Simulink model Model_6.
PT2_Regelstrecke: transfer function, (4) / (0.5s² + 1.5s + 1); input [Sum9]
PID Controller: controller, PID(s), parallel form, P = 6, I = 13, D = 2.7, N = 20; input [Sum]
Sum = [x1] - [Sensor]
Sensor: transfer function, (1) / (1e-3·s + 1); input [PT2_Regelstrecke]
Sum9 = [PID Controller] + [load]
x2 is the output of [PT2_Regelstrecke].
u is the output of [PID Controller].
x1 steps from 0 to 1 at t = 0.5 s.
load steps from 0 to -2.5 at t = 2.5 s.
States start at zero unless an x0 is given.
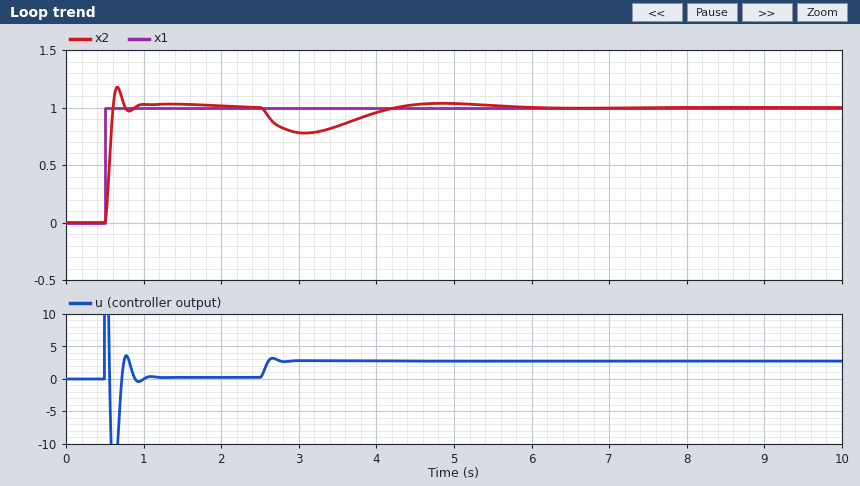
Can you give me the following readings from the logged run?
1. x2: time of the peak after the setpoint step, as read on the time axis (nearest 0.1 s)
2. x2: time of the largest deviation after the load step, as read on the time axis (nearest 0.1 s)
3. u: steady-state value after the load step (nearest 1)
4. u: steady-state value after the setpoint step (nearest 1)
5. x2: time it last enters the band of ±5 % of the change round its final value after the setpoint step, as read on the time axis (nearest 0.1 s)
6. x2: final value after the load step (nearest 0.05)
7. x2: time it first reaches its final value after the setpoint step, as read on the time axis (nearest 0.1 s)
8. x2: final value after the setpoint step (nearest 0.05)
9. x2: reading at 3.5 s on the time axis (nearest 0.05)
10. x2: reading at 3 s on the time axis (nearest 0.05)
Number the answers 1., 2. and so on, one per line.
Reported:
1. 0.7 s
2. 3.1 s
3. 3
4. 0
5. 0.7 s
6. 1.00
7. 0.6 s
8. 1.00
9. 0.85
10. 0.80
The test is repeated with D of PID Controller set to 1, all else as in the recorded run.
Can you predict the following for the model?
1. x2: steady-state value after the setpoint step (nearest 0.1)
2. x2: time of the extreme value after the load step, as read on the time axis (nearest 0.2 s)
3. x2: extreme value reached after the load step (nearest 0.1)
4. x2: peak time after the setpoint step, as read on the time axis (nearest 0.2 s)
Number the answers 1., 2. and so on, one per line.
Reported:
1. 1.0
2. 2.8 s
3. 0.7
4. 0.8 s
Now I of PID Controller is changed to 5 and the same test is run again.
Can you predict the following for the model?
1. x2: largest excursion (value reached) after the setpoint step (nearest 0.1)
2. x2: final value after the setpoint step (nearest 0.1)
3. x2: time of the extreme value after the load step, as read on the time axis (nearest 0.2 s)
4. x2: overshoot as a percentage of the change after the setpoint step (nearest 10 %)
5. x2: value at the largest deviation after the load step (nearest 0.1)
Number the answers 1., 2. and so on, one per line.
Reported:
1. 1.2
2. 1.0
3. 3.4 s
4. 20 %
5. 0.7
